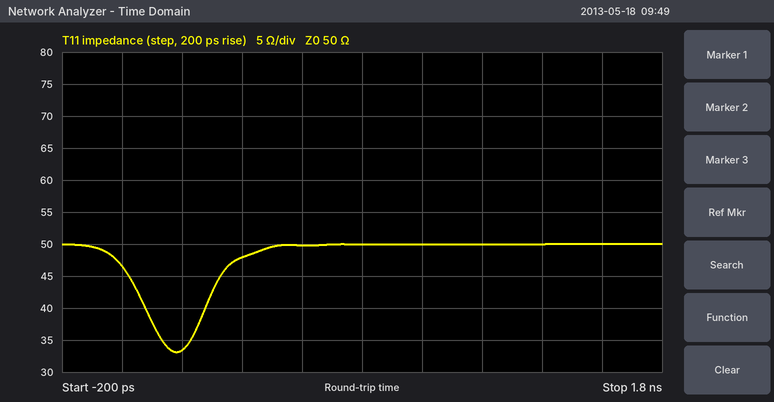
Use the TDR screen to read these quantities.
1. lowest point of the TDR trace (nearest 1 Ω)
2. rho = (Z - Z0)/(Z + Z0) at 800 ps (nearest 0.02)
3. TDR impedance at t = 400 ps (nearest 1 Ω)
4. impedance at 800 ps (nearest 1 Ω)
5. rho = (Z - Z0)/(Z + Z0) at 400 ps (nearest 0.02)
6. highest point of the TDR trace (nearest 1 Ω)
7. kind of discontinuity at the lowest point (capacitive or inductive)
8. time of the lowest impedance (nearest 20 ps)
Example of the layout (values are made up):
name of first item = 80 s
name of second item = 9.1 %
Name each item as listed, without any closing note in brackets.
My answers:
lowest point of the TDR trace = 33 Ω
rho = (Z - Z0)/(Z + Z0) at 800 ps = 0.00
TDR impedance at t = 400 ps = 48 Ω
impedance at 800 ps = 50 Ω
rho = (Z - Z0)/(Z + Z0) at 400 ps = -0.02
highest point of the TDR trace = 50 Ω
kind of discontinuity at the lowest point = capacitive
time of the lowest impedance = 180 ps
